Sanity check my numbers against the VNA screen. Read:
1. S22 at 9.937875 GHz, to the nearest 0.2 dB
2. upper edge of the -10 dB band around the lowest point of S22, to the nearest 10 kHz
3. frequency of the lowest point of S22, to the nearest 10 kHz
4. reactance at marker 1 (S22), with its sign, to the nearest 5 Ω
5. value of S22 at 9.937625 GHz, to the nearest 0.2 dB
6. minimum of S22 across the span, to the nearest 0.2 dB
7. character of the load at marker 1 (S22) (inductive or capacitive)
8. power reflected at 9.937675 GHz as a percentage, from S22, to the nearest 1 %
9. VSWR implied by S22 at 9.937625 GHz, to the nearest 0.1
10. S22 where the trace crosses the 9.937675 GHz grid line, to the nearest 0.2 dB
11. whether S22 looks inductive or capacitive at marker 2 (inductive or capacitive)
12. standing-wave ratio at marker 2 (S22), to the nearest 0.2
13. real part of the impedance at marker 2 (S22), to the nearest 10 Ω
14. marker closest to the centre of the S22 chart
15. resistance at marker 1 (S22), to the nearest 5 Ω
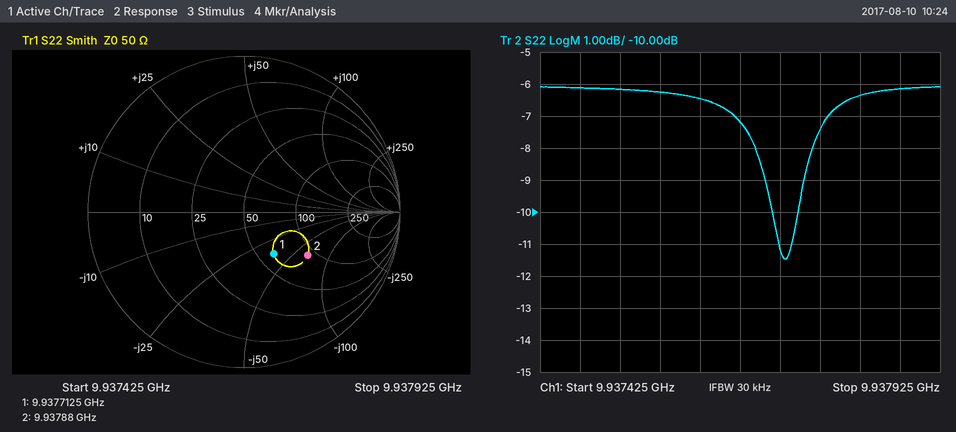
-6.2 dB
9.93775 GHz
9.93773 GHz
-35 Ω
-6.4 dB
-11.4 dB
capacitive
19 %
2.8
-7.2 dB
capacitive
3.0
90 Ω
marker 1
60 Ω
